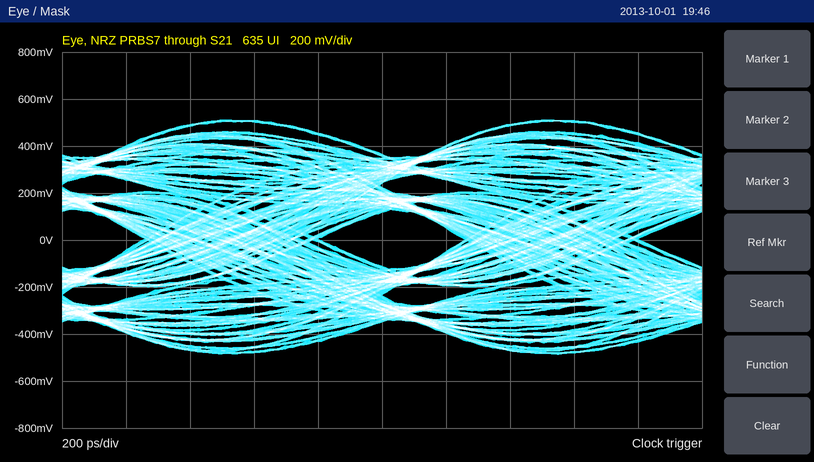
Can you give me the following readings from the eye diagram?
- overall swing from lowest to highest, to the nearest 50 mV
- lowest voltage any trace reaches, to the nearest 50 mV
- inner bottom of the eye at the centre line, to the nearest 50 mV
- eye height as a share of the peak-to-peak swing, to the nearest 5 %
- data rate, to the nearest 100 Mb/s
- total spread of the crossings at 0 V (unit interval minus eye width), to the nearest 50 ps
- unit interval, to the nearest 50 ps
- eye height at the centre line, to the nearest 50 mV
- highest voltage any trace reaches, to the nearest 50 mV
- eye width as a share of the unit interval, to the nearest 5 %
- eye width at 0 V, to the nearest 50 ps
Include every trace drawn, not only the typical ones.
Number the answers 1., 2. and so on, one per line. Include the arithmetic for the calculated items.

1. 1.00 V
2. -500 mV
3. -100 mV
4. 250 mV / 1.00 V ≈ 25 %
5. 1.0 Gb/s
6. 550 ps
7. 1.00 ns
8. 250 mV
9. 500 mV
10. 450 ps / 1.00 ns ≈ 45 %
11. 450 ps
